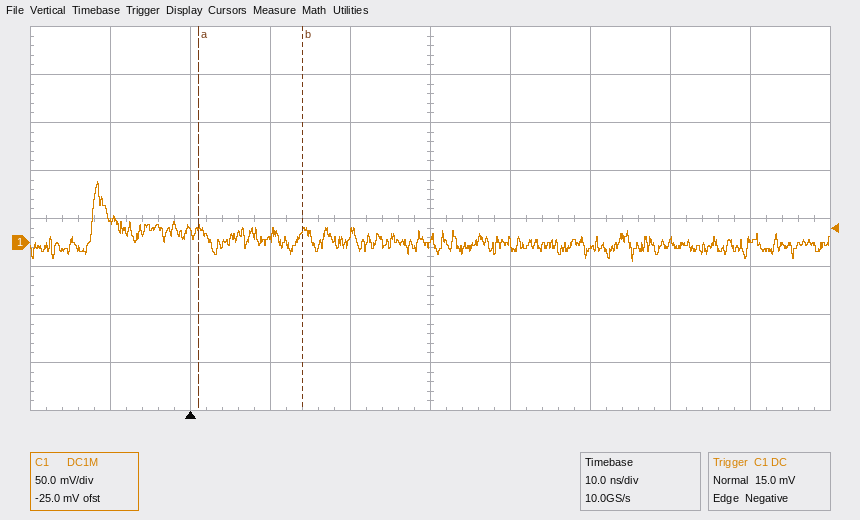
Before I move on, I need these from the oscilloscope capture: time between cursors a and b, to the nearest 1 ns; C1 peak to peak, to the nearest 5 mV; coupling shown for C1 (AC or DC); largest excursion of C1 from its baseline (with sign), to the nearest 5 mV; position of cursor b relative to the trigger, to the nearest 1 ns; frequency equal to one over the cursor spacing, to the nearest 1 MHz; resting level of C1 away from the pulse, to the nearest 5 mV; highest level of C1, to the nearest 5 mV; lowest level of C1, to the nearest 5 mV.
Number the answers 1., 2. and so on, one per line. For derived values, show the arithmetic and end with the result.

1. 13 ns
2. 65 mV − (-20 mV) = 85 mV
3. DC
4. 65 mV − (0 mV) = +65 mV
5. +14 ns
6. 1 / 13 ns ≈ 77 MHz
7. 0 mV
8. 65 mV
9. -20 mV
